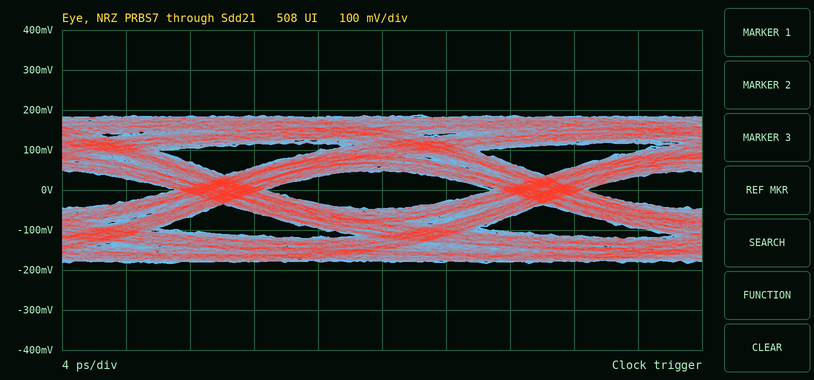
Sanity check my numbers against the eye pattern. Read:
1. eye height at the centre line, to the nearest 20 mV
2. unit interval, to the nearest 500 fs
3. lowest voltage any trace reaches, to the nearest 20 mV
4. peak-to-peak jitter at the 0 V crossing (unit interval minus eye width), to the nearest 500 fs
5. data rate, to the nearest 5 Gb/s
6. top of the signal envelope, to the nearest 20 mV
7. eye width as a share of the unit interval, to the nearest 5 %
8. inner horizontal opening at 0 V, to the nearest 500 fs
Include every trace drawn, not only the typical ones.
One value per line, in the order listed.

100 mV
20.0 ps
-180 mV
6.0 ps
50 Gb/s
180 mV
70 %
14.0 ps
